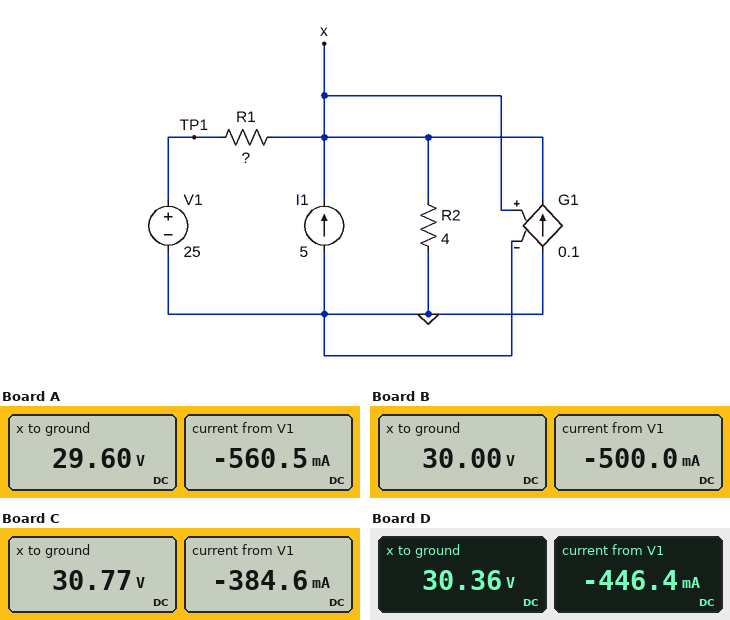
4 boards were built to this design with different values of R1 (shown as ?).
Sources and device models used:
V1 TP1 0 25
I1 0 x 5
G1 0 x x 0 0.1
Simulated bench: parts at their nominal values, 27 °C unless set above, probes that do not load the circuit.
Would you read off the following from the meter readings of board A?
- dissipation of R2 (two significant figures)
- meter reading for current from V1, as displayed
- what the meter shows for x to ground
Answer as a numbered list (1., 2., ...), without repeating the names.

1. 220 W
2. -560.5 mA
3. 29.60 V
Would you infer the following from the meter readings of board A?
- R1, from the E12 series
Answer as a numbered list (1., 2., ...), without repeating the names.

1. 8.2 Ω
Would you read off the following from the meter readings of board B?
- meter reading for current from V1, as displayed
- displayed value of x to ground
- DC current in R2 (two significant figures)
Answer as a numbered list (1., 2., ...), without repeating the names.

1. -500.0 mA
2. 30.00 V
3. 7.5 A
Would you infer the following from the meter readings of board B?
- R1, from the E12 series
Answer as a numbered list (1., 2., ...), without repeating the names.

1. 10 Ω
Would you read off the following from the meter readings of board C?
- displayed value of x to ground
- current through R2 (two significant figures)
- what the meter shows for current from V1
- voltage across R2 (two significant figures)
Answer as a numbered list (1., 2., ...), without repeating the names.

1. 30.77 V
2. 7.7 A
3. -384.6 mA
4. 31 V
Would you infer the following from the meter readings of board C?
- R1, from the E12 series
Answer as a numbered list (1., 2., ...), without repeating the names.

1. 15 Ω
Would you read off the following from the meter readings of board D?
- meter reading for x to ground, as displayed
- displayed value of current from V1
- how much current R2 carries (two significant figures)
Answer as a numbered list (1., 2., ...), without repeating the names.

1. 30.36 V
2. -446.4 mA
3. 7.6 A
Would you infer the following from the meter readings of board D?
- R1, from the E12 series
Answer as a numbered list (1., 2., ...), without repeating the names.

1. 12 Ω
